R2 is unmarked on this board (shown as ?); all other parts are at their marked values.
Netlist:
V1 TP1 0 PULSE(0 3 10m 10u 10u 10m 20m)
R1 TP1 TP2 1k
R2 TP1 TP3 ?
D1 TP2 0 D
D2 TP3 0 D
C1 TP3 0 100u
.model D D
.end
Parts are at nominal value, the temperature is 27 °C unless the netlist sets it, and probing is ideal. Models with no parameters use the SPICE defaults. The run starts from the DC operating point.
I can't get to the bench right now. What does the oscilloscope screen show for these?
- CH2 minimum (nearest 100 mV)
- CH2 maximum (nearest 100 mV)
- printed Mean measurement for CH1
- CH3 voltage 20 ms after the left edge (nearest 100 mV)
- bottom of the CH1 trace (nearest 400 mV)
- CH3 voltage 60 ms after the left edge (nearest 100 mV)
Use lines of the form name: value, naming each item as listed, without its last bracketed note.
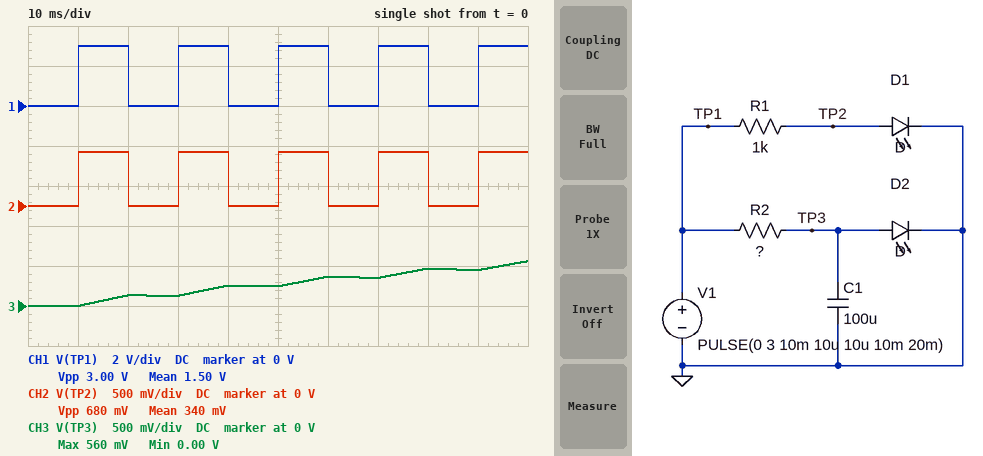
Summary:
CH2 minimum: 0 V
CH2 maximum: 700 mV
printed Mean measurement for CH1: 1.50 V
CH3 voltage 20 ms after the left edge: 100 mV
bottom of the CH1 trace: 0 V
CH3 voltage 60 ms after the left edge: 400 mV
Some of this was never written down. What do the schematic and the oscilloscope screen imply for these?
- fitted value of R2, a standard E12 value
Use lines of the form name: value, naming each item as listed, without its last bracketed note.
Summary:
fitted value of R2, a standard E12 value: 2.2 kΩ
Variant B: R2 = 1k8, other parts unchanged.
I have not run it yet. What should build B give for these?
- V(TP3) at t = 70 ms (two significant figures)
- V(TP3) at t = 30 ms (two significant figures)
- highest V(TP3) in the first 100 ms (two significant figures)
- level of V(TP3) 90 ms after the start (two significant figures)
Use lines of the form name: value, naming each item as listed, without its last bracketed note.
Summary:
V(TP3) at t = 70 ms: 410 mV
V(TP3) at t = 30 ms: 150 mV
highest V(TP3) in the first 100 ms: 640 mV
level of V(TP3) 90 ms after the start: 520 mV
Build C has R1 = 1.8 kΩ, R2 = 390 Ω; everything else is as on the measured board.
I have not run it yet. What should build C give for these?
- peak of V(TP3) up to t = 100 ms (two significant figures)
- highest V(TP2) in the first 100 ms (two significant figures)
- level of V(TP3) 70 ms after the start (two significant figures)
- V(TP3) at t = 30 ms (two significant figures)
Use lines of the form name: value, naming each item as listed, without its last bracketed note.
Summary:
peak of V(TP3) up to t = 100 ms: 700 mV
highest V(TP2) in the first 100 ms: 660 mV
level of V(TP3) 70 ms after the start: 510 mV
V(TP3) at t = 30 ms: 500 mV
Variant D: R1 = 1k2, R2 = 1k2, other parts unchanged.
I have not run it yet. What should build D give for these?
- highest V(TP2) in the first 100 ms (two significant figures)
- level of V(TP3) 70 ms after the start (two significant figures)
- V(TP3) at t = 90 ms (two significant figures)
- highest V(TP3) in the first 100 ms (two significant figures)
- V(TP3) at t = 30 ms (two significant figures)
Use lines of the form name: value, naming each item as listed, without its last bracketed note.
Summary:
highest V(TP2) in the first 100 ms: 670 mV
level of V(TP3) 70 ms after the start: 560 mV
V(TP3) at t = 90 ms: 580 mV
highest V(TP3) in the first 100 ms: 670 mV
V(TP3) at t = 30 ms: 220 mV
